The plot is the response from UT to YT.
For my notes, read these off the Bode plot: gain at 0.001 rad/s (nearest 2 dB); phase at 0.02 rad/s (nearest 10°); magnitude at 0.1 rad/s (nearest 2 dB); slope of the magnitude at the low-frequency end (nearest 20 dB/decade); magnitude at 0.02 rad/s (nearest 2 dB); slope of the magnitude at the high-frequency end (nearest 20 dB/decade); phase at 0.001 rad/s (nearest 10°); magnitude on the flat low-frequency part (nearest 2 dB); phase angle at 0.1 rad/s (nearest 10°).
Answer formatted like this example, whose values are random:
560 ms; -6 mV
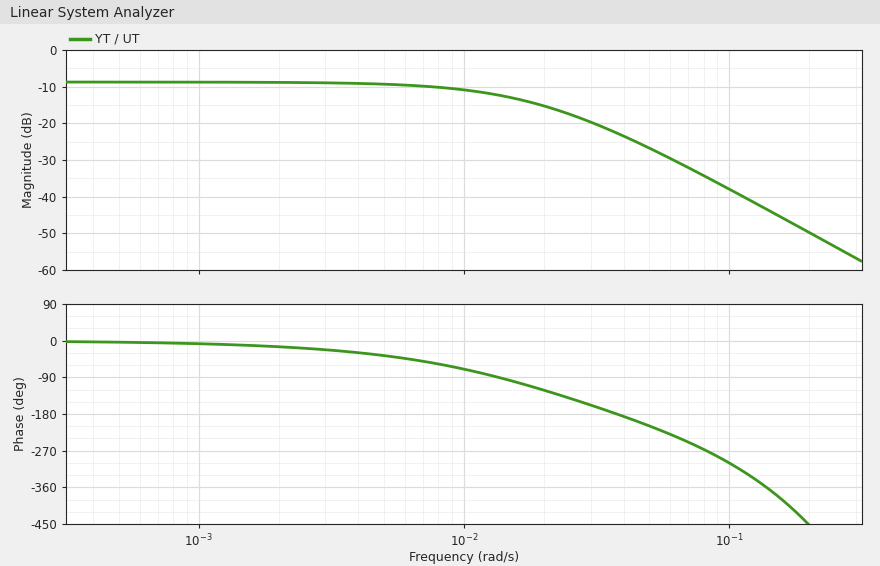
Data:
-8 dB; -120°; -38 dB; 0 dB/decade; -16 dB; -40 dB/decade; -10°; -8 dB; -300°
